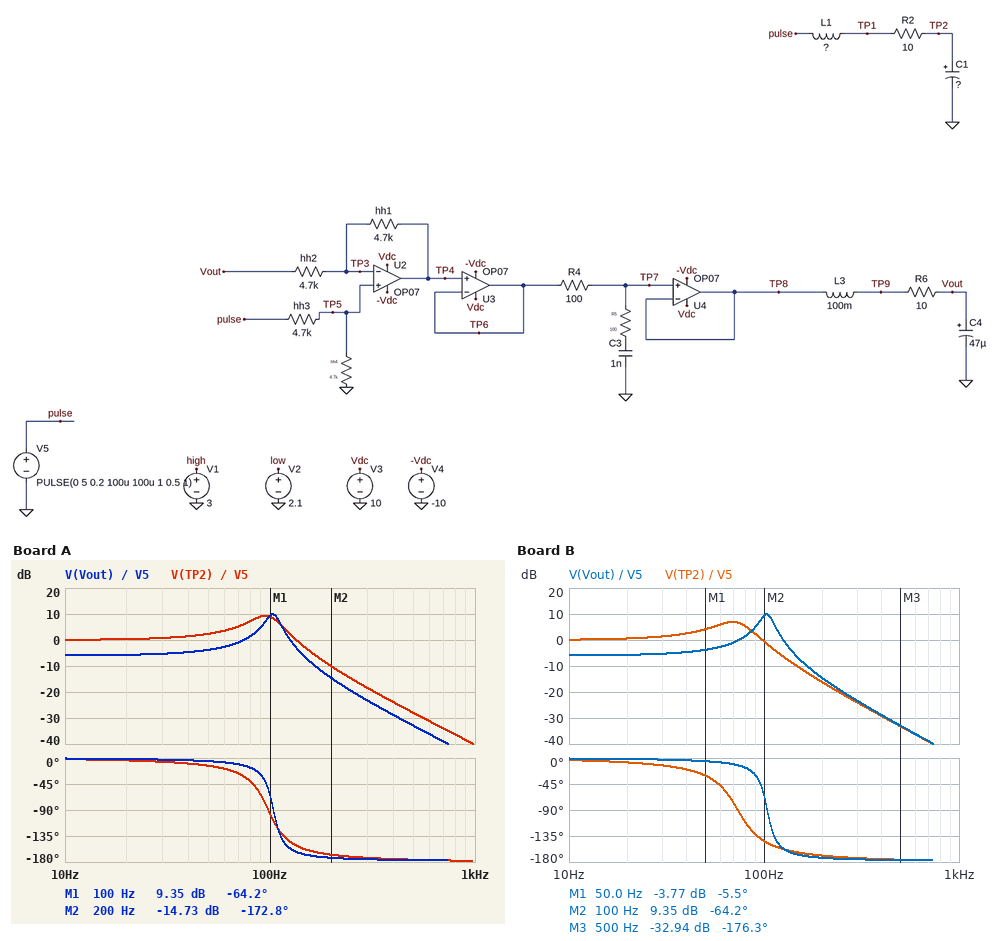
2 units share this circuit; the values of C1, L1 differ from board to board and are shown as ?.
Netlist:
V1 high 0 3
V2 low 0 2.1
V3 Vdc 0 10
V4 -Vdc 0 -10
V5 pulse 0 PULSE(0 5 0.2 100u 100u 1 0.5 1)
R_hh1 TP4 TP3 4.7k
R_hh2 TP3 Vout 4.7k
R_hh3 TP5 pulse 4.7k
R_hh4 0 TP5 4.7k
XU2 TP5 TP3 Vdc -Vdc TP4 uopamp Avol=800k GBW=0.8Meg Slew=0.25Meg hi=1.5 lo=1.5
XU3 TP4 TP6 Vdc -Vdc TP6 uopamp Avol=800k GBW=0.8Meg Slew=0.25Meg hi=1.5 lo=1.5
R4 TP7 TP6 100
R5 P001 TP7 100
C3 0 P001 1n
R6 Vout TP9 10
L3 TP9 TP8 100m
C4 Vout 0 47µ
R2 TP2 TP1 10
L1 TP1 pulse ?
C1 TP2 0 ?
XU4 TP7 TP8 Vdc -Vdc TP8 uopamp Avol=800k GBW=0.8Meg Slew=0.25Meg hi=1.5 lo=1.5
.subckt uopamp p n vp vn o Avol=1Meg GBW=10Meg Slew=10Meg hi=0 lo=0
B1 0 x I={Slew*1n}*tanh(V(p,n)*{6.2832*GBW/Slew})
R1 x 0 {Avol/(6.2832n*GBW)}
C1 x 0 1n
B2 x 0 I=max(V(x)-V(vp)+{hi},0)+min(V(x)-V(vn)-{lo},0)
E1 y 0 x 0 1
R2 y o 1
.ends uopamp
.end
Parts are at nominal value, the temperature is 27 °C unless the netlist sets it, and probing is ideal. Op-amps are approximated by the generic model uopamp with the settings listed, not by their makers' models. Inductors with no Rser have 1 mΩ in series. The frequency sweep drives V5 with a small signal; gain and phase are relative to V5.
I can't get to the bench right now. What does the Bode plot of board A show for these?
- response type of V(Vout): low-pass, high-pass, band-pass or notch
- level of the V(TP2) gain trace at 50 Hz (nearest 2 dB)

low-pass
2 dB
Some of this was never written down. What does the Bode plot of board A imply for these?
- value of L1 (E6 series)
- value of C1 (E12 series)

47 mH
56 µF
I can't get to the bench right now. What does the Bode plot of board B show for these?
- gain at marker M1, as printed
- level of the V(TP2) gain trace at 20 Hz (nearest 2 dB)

-3.77 dB
0 dB
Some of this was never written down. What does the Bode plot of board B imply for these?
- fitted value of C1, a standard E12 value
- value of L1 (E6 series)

100 µF
47 mH
